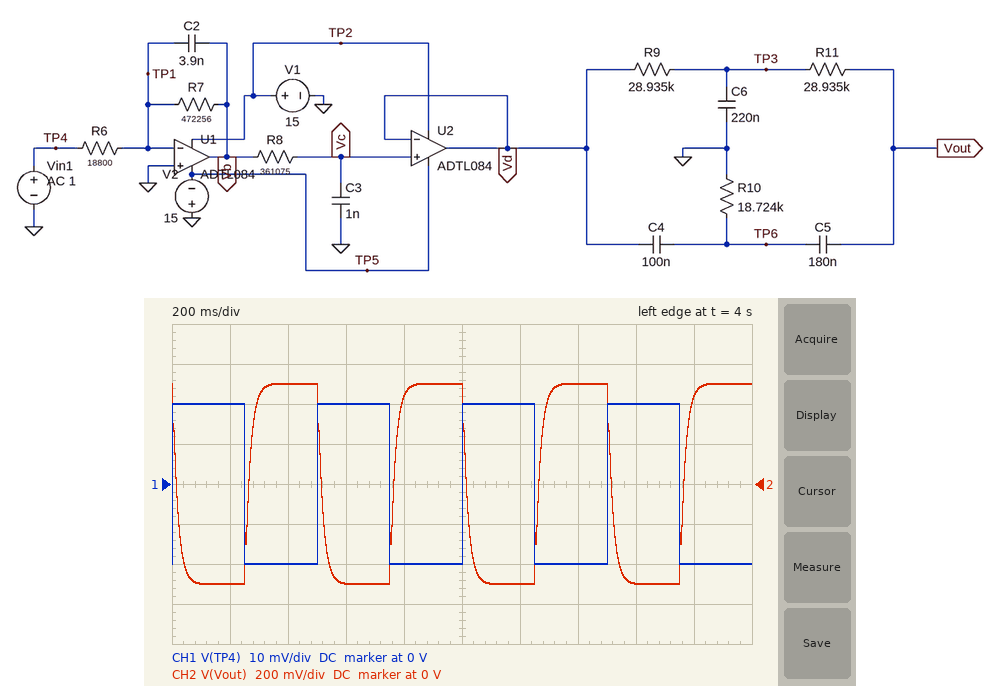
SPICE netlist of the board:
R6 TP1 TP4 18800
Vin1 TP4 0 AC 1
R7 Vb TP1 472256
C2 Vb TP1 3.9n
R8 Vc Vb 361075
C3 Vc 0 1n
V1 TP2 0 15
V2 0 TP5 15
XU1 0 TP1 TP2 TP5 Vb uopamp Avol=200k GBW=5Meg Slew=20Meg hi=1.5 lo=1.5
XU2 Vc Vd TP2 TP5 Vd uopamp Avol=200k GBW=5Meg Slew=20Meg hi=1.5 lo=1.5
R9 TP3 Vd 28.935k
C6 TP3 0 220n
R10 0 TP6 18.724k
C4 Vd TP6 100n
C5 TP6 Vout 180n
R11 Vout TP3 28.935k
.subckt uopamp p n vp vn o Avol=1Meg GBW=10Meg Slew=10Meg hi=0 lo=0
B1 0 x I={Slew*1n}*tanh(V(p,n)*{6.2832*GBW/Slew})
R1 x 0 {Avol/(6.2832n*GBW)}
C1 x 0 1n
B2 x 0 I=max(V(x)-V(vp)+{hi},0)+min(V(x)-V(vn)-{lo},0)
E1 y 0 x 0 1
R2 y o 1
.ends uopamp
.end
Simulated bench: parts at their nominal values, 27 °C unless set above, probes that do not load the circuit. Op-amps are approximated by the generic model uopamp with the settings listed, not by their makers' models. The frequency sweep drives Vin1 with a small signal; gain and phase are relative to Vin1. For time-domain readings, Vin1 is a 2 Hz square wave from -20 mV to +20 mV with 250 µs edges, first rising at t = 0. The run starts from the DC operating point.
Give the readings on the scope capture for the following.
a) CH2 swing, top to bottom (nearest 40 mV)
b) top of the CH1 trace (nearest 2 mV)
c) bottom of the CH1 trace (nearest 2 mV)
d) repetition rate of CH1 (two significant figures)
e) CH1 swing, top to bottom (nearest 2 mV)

1.00 V
20 mV
-20 mV
2.0 Hz
40 mV
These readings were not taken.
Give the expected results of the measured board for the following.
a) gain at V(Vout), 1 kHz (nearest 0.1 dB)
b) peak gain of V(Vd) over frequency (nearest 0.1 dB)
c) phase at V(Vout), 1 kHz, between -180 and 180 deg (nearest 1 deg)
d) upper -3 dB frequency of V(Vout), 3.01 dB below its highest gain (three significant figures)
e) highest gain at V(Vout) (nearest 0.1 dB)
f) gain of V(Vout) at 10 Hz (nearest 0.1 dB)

-1.3 dB
28.0 dB
38 deg
8.42 Hz
28.0 dB
24.1 dB
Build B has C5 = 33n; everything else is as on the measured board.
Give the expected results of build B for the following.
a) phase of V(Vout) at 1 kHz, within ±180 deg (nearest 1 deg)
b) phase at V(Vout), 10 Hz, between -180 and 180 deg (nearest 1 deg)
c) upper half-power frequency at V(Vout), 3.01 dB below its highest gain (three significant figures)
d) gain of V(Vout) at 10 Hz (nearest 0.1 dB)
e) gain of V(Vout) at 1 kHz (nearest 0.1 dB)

46 deg
144 deg
17.8 Hz
26.9 dB
-1.6 dB
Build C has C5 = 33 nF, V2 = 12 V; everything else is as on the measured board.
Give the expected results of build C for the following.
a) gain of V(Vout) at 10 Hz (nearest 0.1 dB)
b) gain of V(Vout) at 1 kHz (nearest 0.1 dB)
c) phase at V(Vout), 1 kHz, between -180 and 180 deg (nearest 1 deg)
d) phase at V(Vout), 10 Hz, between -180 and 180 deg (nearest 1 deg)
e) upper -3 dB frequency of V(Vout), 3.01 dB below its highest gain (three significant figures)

26.9 dB
-1.6 dB
46 deg
144 deg
17.8 Hz
